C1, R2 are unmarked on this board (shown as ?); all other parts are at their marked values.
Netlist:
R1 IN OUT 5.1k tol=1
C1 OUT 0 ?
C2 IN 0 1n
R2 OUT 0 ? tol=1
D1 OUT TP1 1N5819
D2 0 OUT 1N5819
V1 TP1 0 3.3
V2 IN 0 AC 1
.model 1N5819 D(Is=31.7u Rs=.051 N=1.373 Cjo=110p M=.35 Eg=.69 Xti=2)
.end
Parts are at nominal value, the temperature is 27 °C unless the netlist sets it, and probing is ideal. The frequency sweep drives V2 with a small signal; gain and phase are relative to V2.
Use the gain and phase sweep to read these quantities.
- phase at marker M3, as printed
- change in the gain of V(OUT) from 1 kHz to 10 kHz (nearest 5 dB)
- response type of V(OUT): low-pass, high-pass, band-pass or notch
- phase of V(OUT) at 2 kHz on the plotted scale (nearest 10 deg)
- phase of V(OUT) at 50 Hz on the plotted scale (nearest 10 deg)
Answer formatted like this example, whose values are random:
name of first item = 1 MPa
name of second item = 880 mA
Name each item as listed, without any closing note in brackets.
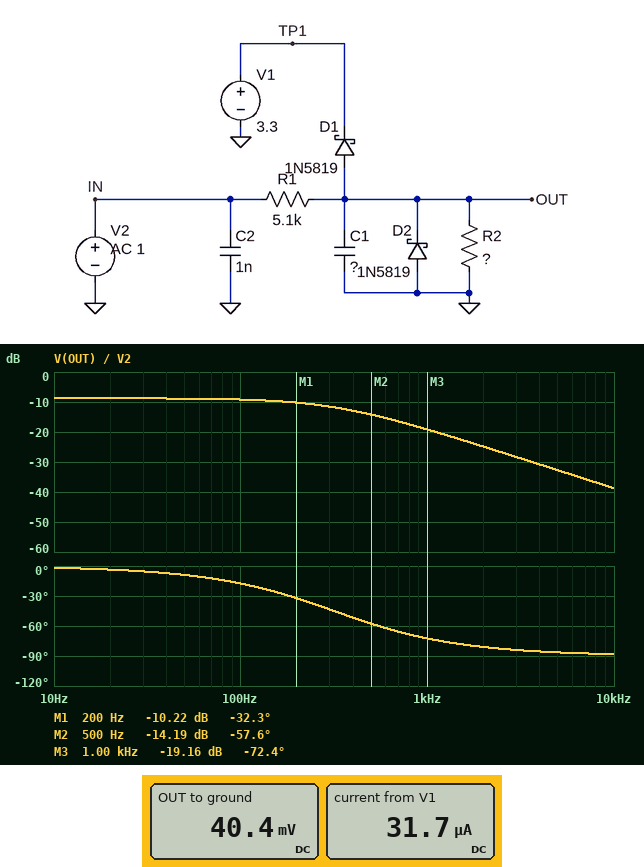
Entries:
phase at marker M3, as printed = -72.4 deg
change in the gain of V(OUT) from 1 kHz to 10 kHz = -20 dB
response type of V(OUT): low-pass, high-pass, band-pass or notch = low-pass
phase of V(OUT) at 2 kHz on the plotted scale = -80 deg
phase of V(OUT) at 50 Hz on the plotted scale = -10 deg
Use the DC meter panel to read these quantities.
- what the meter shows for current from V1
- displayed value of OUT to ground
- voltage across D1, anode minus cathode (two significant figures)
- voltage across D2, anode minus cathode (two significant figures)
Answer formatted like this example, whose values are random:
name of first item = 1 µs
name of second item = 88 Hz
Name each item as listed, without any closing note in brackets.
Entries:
what the meter shows for current from V1 = 31.7 µA
displayed value of OUT to ground = 40.4 mV
voltage across D1, anode minus cathode = -3.3 V
voltage across D2, anode minus cathode = -40 mV
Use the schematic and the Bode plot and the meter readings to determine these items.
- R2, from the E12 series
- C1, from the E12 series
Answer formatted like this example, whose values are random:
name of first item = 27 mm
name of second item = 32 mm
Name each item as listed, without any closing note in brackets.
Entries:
R2, from the E12 series = 18 kΩ
C1, from the E12 series = 270 nF
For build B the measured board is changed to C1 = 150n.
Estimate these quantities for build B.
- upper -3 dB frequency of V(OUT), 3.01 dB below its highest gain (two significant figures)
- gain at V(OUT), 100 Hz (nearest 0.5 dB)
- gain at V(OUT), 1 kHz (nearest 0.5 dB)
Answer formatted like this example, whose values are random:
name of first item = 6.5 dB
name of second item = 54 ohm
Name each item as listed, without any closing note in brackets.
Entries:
upper -3 dB frequency of V(OUT), 3.01 dB below its highest gain = 570 Hz
gain at V(OUT), 100 Hz = -9.0 dB
gain at V(OUT), 1 kHz = -15.0 dB
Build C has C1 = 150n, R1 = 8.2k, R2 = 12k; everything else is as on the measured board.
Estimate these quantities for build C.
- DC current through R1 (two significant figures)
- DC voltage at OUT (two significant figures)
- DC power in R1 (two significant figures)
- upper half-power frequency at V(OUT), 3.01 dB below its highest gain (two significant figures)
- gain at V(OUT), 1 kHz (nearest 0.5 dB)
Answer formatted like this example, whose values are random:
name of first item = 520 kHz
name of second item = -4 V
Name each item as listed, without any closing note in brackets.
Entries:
DC current through R1 = 5.4 µA
DC voltage at OUT = 44 mV
DC power in R1 = 240 nW
upper half-power frequency at V(OUT), 3.01 dB below its highest gain = 490 Hz
gain at V(OUT), 1 kHz = -18.5 dB
